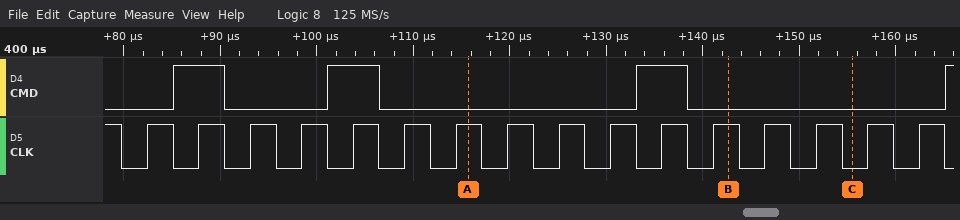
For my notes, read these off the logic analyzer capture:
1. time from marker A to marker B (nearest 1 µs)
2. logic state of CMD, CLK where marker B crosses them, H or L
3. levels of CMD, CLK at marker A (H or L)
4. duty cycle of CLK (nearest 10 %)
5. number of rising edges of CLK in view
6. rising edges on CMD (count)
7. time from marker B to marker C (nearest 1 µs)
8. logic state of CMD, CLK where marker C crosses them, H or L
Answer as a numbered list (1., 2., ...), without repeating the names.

1. 27 µs
2. CMD=L, CLK=H
3. CMD=L, CLK=H
4. 50 %
5. 16
6. 4
7. 13 µs
8. CMD=L, CLK=L
